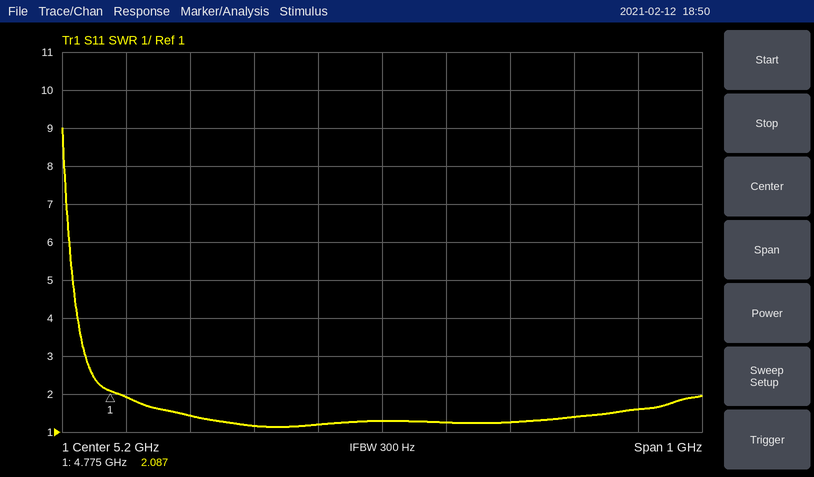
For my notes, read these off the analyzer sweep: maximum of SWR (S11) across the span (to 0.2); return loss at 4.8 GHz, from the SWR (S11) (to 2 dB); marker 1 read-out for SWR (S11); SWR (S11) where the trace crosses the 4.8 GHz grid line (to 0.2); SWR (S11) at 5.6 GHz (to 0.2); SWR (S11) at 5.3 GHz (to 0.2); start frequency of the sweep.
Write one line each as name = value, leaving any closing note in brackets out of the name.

maximum of SWR (S11) across the span = 9.0
return loss at 4.8 GHz, from the SWR (S11) = 10 dB
marker 1 read-out for SWR = 2.087
SWR (S11) where the trace crosses the 4.8 GHz grid line = 2.0
SWR (S11) at 5.6 GHz = 1.6
SWR (S11) at 5.3 GHz = 1.2
start frequency of the sweep = 4.7 GHz
